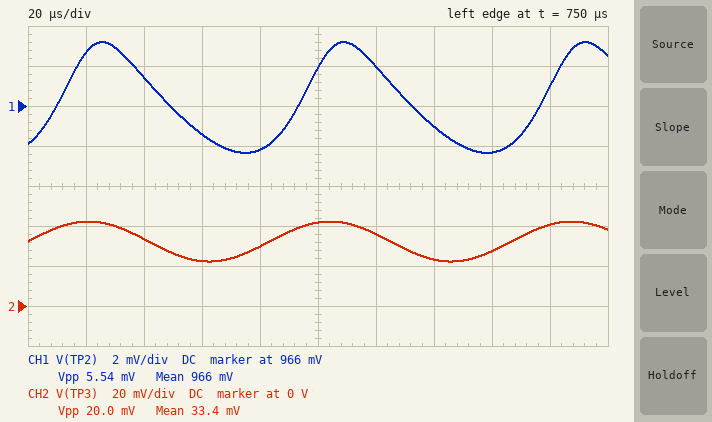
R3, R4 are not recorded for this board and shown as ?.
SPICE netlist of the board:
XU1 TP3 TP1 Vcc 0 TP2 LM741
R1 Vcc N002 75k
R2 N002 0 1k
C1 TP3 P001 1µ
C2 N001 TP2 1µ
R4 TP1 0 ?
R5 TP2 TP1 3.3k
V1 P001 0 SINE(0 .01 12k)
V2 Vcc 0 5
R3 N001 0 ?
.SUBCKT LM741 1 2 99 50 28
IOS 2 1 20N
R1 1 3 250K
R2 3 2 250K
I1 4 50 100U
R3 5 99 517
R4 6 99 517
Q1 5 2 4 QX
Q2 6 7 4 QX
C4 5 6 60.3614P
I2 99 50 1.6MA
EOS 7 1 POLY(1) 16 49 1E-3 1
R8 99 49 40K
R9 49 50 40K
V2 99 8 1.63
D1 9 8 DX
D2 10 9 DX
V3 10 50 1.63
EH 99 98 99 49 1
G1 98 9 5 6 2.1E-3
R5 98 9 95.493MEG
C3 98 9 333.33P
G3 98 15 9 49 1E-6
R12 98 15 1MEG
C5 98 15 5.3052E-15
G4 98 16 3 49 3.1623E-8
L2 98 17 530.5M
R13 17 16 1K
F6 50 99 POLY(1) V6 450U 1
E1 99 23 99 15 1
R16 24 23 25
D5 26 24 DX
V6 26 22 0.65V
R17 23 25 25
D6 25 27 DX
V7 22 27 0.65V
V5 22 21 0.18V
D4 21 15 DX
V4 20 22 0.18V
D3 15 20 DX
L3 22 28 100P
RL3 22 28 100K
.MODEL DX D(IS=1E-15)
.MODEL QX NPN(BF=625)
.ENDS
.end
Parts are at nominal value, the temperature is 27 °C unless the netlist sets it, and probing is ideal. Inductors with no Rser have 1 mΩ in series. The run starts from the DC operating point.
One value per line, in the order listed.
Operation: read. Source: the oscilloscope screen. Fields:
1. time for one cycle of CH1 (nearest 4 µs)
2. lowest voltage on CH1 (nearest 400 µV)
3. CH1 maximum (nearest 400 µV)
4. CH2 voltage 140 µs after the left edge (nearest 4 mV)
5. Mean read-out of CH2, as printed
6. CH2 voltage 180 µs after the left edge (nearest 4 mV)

84 µs
963.6 mV
969.2 mV
24 mV
33.4 mV
40 mV
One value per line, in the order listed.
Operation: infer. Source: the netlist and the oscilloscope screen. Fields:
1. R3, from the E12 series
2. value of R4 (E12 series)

15 Ω
180 Ω
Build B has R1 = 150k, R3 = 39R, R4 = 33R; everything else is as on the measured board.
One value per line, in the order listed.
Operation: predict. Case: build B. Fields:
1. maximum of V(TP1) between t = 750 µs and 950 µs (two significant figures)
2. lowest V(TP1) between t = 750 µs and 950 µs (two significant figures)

9.6 mV
9.5 mV
